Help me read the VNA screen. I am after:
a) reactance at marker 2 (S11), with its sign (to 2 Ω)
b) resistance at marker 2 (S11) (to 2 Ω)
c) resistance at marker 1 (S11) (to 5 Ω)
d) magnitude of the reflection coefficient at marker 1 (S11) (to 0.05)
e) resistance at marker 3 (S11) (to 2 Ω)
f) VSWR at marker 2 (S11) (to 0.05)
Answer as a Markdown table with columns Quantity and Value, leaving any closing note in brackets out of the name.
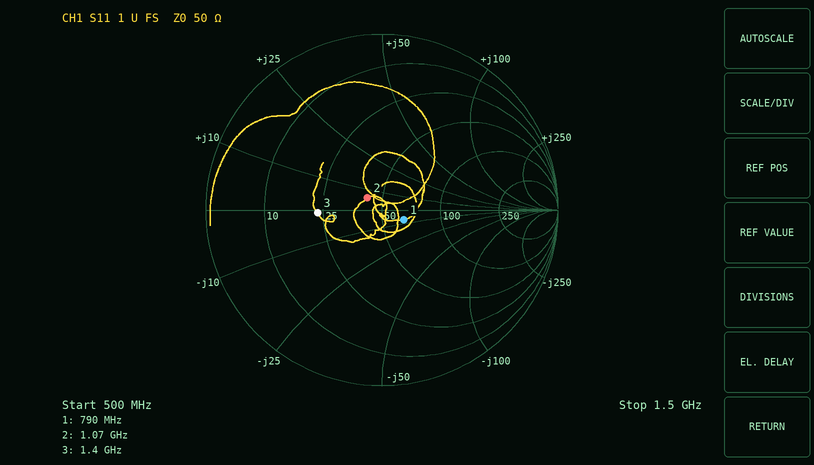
| Quantity | Value |
|---|---|
| reactance at marker 2 (S11), with its sign | +6 Ω |
| resistance at marker 2 (S11) | 42 Ω |
| resistance at marker 1 (S11) | 65 Ω |
| magnitude of the reflection coefficient at marker 1 (S11) | 0.15 |
| resistance at marker 3 (S11) | 24 Ω |
| VSWR at marker 2 (S11) | 1.25 |
